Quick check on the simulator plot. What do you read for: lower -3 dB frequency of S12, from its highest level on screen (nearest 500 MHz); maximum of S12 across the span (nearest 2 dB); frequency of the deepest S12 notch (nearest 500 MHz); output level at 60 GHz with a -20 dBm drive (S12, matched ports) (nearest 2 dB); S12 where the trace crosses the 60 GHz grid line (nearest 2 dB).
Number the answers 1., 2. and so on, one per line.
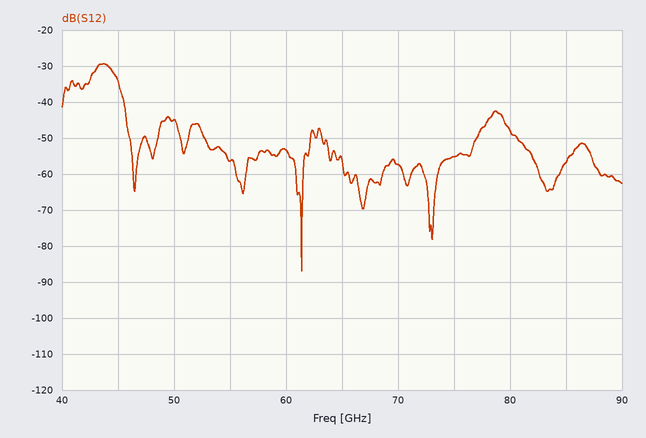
1. 42.5 GHz
2. -30 dB
3. 61.5 GHz
4. -74 dBm
5. -54 dB
